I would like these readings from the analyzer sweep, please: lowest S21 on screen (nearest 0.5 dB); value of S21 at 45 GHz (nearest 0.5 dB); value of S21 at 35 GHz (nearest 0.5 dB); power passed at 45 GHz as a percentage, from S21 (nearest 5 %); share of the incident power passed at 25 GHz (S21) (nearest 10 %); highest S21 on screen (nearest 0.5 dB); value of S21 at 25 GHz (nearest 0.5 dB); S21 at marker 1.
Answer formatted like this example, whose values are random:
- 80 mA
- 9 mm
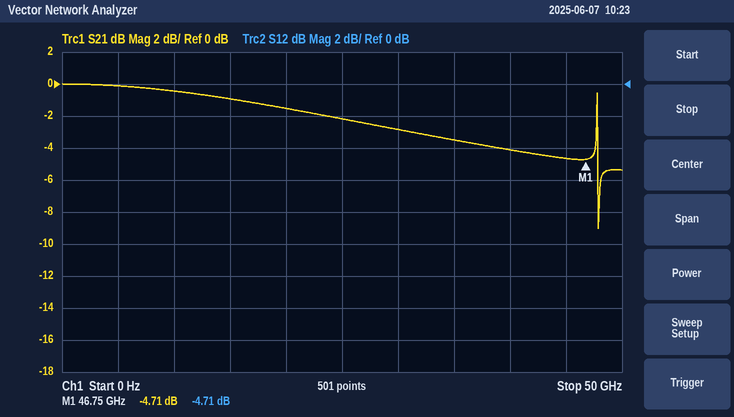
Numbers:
- -9.0 dB
- -4.5 dB
- -3.5 dB
- 35 %
- 60 %
- 0.0 dB
- -2.0 dB
- -4.71 dB
